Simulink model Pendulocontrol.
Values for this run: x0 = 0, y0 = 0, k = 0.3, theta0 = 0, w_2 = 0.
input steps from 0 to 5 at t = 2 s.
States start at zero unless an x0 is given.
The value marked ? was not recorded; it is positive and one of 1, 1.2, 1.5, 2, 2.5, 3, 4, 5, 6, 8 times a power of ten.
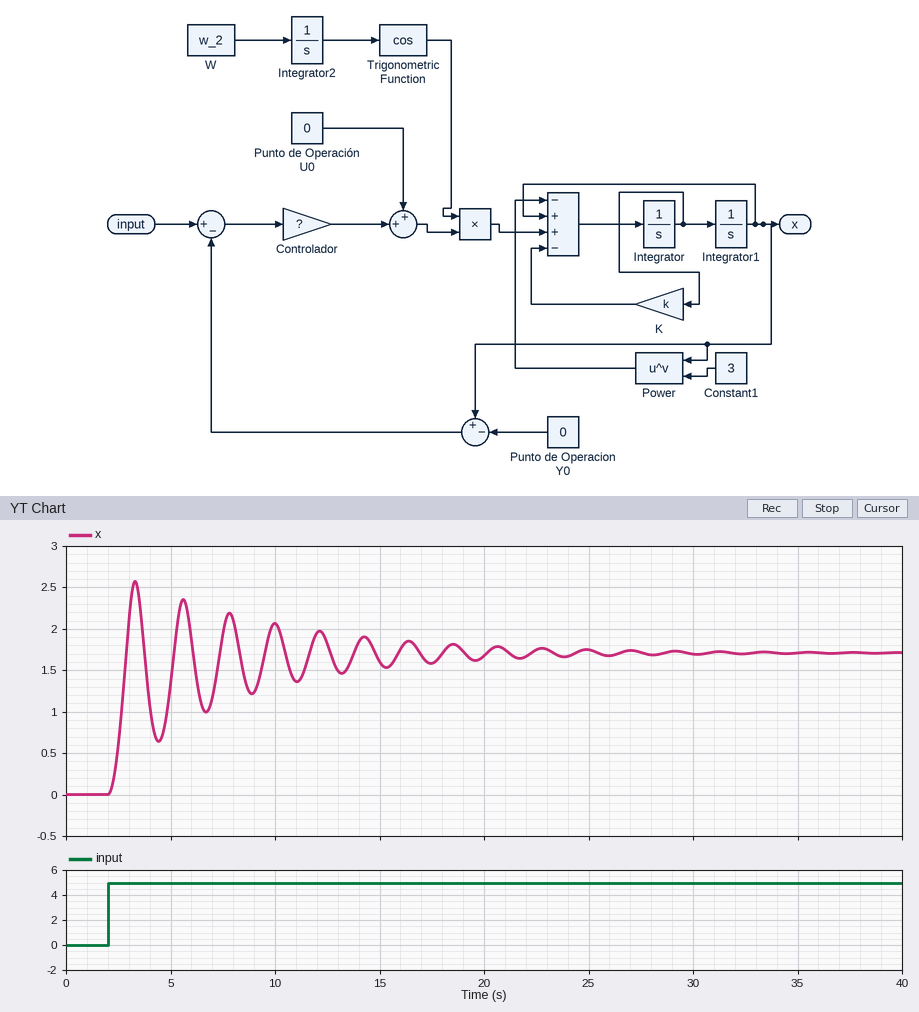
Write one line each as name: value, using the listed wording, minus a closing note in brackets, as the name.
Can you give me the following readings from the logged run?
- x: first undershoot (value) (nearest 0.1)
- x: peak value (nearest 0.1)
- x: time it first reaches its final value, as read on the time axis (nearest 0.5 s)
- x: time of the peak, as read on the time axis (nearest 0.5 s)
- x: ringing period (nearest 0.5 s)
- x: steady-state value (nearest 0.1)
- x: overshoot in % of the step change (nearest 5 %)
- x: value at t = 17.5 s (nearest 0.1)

x: first undershoot (value): 0.6
x: peak value: 2.6
x: time it first reaches its final value, as read on the time axis: 3.0 s
x: time of the peak, as read on the time axis: 3.5 s
x: ringing period: 2.5 s
x: steady-state value: 1.7
x: overshoot in % of the step change: 50 %
x: value at t = 17.5 s: 1.6
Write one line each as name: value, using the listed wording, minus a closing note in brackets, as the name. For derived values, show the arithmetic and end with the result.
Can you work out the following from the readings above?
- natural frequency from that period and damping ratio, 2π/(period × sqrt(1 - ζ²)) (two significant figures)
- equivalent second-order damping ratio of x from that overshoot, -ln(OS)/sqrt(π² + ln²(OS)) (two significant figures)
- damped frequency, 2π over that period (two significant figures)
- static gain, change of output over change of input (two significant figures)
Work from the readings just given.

natural frequency from that period and damping ratio, 2π/(period × sqrt(1 - ζ²)): 2π / (2.5 × sqrt(1 - 0.22²)) = 2.6 rad/s
equivalent second-order damping ratio of x from that overshoot, -ln(OS)/sqrt(π² + ln²(OS)): ln(0.5) = -0.693; 0.693 / sqrt(9.870 + 0.480) = 0.22
damped frequency, 2π over that period: 2π / 2.5 = 2.5 rad/s
static gain, change of output over change of input: (1.7 - 0) / (5 - 0) = 0.34
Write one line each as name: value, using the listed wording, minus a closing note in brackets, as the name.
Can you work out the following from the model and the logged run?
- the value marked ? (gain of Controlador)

the value marked ?: 1
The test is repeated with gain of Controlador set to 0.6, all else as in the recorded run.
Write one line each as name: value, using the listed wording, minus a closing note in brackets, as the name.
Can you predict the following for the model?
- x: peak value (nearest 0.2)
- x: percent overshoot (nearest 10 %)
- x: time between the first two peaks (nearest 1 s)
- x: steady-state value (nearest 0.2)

x: peak value: 2.2
x: percent overshoot: 50 %
x: time between the first two peaks: 3 s
x: steady-state value: 1.6
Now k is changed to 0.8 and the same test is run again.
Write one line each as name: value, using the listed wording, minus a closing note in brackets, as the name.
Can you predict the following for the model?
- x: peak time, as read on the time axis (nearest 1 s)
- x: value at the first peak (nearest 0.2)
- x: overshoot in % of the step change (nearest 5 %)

x: peak time, as read on the time axis: 3 s
x: value at the first peak: 2.4
x: overshoot in % of the step change: 40 %
